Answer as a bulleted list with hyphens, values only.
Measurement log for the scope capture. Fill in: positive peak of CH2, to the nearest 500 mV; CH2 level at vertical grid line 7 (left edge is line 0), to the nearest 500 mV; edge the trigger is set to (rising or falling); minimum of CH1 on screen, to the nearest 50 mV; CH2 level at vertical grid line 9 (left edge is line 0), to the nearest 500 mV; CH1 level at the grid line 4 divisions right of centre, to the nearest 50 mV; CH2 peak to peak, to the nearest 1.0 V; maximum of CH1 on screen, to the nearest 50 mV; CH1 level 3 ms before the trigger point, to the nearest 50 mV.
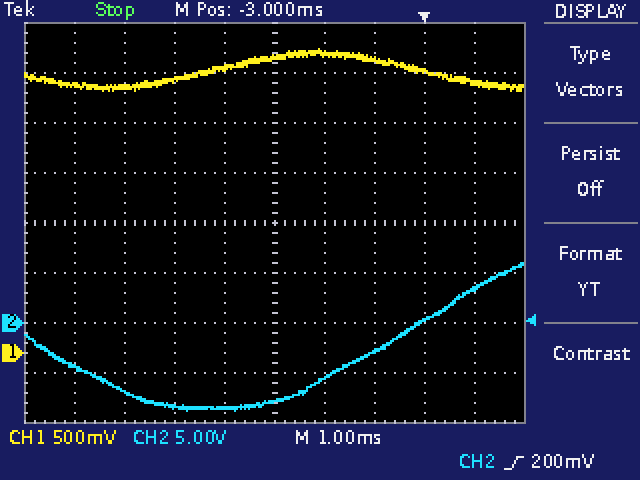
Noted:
- 6.0 V
- -3.0 V
- rising
- 2.60 V
- 3.5 V
- 2.70 V
- 15.0 V
- 3.05 V
- 2.95 V
